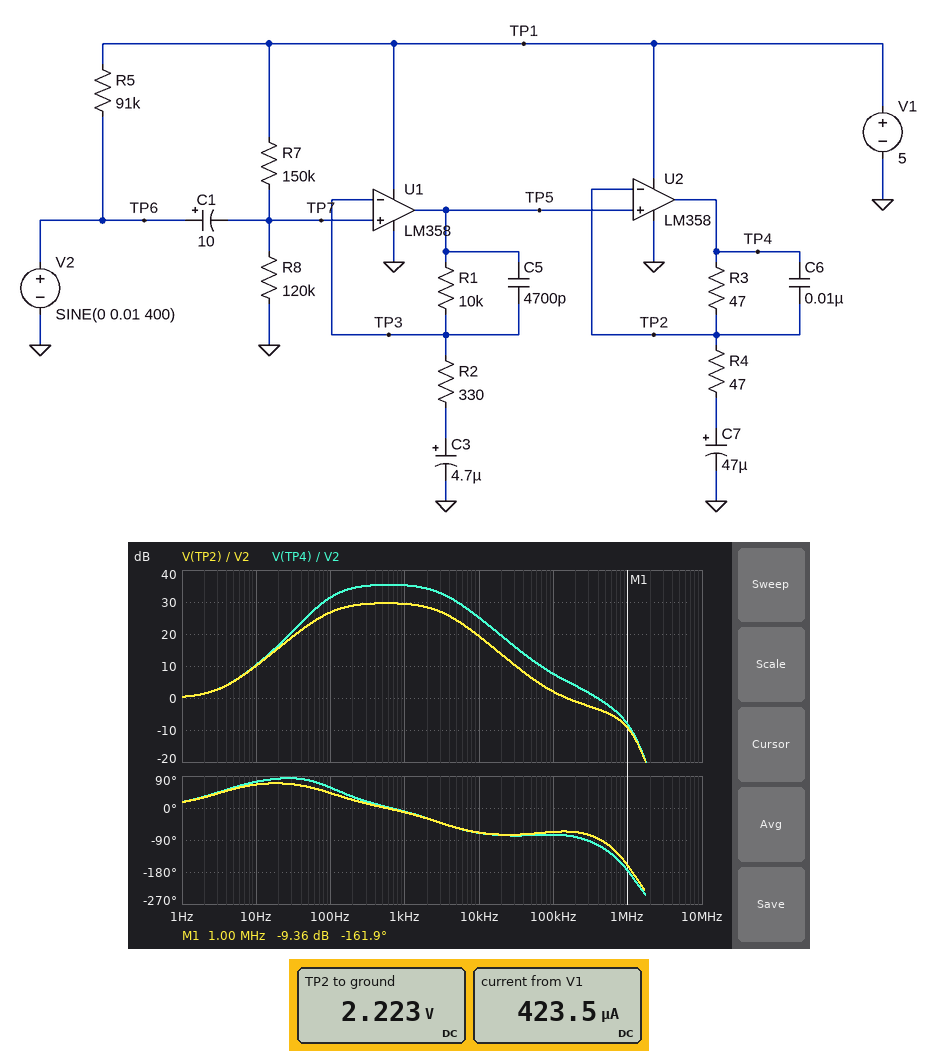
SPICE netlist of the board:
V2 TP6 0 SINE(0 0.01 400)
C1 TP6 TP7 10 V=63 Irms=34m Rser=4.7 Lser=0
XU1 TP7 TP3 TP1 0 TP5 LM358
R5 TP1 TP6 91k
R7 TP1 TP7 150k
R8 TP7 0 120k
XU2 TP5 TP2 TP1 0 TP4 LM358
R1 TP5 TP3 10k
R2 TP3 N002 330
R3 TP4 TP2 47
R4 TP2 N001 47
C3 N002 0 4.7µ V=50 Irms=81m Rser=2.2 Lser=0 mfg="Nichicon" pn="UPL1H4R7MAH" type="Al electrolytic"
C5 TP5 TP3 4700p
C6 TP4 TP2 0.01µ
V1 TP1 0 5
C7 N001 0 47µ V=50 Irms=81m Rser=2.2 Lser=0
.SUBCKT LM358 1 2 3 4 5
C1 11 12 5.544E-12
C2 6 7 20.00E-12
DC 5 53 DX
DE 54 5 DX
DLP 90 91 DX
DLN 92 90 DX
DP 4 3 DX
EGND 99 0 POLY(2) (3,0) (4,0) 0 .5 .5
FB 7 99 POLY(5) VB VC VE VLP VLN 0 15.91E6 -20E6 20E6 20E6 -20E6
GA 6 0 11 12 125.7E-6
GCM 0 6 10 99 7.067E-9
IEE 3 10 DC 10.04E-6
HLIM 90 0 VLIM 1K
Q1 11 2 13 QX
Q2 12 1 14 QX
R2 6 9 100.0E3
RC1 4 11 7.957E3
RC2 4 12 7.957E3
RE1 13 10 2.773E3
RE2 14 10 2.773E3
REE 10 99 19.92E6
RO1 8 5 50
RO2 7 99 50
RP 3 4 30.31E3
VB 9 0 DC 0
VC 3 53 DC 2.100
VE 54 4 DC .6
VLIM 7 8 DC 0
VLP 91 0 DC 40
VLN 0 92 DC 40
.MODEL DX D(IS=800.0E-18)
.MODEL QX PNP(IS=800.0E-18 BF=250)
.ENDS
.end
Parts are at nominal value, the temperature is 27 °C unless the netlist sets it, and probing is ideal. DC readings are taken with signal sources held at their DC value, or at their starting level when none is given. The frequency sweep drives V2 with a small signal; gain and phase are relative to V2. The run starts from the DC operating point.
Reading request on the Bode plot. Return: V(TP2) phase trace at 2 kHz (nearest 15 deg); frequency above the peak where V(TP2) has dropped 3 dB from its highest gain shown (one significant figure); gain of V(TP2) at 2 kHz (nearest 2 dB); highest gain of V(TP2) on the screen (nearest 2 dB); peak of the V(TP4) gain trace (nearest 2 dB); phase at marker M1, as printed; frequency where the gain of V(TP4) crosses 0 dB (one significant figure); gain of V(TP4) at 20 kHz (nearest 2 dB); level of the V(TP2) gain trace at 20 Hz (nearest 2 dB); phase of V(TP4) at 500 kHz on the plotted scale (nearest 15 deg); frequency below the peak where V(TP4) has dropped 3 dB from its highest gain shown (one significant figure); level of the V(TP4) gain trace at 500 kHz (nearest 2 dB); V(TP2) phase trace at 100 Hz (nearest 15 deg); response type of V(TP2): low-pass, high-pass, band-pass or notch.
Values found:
-30 deg
3 kHz
28 dB
30 dB
36 dB
-161.9 deg
400 kHz
20 dB
16 dB
-120 deg
100 Hz
-2 dB
45 deg
band-pass
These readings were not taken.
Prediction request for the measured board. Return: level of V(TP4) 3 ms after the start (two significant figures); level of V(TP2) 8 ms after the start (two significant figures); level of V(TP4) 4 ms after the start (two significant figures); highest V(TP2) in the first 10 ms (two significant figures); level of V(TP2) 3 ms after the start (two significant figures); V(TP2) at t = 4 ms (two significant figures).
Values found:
2.8 V
2.5 V
1.8 V
2.5 V
2.5 V
2.0 V
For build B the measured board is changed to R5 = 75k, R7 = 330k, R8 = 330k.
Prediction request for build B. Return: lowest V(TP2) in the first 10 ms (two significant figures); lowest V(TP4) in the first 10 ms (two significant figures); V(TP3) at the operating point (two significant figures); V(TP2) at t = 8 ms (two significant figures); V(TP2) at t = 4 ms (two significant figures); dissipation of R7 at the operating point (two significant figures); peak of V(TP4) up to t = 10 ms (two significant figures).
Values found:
2.2 V
1.9 V
2.5 V
2.8 V
2.3 V
19 µW
3.1 V
